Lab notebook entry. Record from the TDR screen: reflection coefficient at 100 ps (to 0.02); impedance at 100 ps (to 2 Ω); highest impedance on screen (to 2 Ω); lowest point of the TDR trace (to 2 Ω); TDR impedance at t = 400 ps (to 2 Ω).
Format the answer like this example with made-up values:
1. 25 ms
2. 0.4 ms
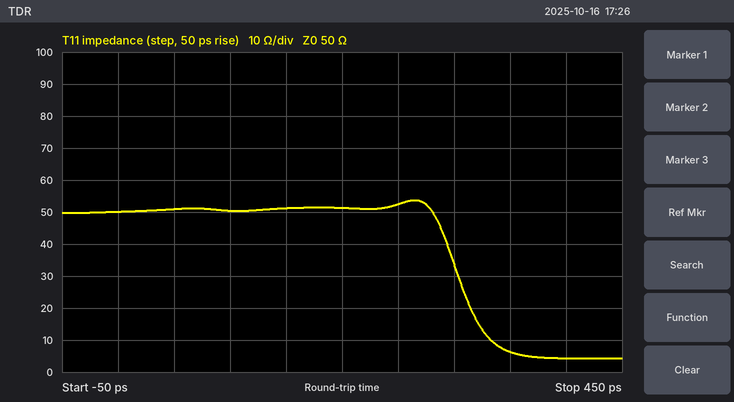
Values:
1. 0.00
2. 50 Ω
3. 54 Ω
4. 4 Ω
5. 4 Ω
